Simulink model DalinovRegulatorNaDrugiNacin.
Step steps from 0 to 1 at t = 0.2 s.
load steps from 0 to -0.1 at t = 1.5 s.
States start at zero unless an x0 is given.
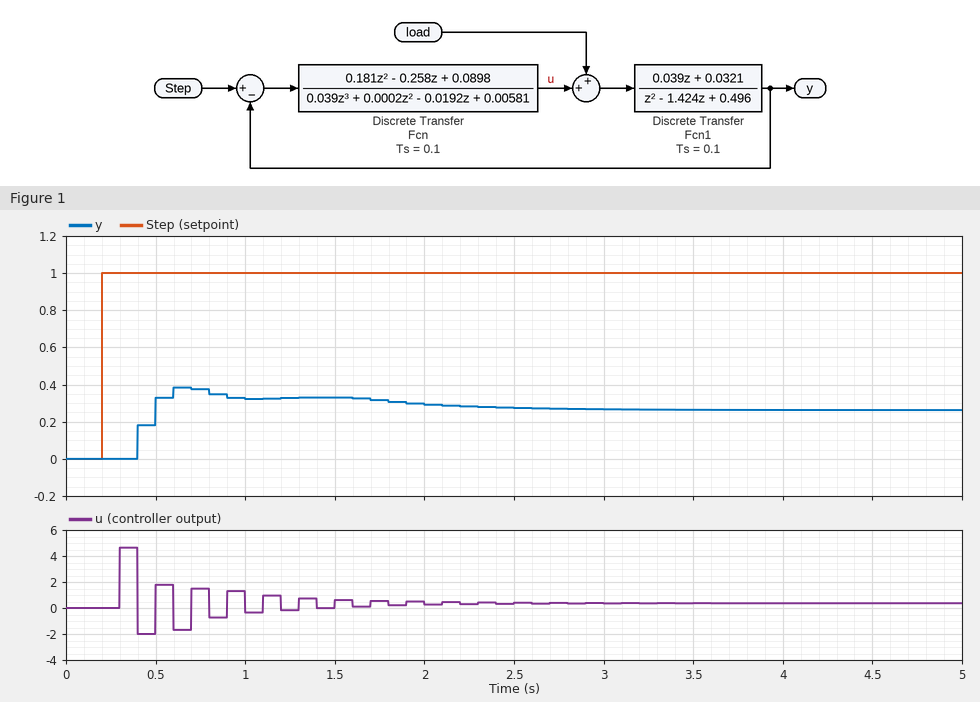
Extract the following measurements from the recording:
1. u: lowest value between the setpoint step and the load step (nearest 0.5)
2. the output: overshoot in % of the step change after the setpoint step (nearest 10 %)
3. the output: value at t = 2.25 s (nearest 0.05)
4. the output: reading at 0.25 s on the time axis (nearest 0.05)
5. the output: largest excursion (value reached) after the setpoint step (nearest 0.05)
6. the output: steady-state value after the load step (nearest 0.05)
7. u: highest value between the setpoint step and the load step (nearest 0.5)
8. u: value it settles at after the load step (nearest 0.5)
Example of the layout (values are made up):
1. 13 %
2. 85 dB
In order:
1. -2.0
2. 20 %
3. 0.30
4. 0.00
5. 0.40
6. 0.25
7. 4.5
8. 0.5
